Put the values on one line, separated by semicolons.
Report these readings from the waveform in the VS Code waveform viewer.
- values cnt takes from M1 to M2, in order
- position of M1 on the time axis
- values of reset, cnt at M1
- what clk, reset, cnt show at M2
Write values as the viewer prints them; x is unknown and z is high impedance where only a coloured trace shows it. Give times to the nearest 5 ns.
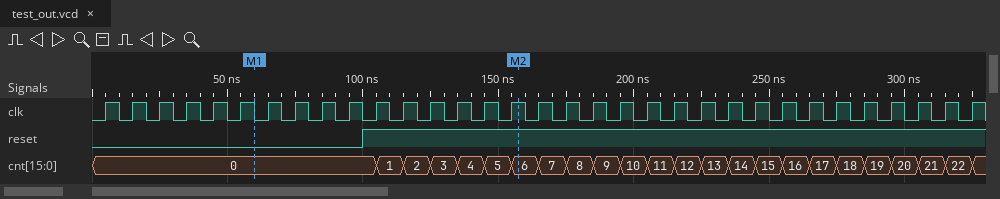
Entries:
0, 1, 2, 3, 4, 5, 6; 60 ns; reset=0, cnt=0; clk=1, reset=1, cnt=6
